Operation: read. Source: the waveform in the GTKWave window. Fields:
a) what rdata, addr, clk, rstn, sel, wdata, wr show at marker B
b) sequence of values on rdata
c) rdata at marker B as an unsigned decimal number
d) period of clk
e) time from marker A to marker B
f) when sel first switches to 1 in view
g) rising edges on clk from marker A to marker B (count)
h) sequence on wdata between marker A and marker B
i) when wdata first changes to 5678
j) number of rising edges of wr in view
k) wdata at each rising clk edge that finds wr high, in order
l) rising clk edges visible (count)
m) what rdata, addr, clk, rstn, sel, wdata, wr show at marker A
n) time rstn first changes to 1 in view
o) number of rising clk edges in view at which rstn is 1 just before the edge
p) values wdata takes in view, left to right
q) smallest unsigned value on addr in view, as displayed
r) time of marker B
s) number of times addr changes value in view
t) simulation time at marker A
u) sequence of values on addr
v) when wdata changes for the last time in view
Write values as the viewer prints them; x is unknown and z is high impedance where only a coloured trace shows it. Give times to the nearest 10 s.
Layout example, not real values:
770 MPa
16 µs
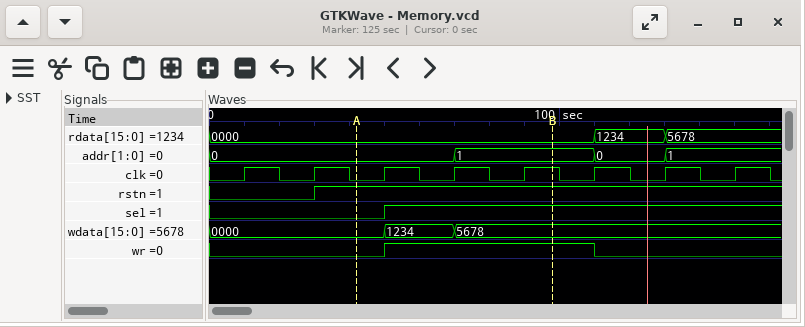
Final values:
rdata=0000, addr=1, clk=1, rstn=1, sel=1, wdata=5678, wr=1
0000, 1234, 5678
0
20 s
60 s
50 s
3
0000, 1234, 5678
70 s
1
1234, 5678, 5678
8
rdata=0000, addr=0, clk=0, rstn=1, sel=0, wdata=0000, wr=0
30 s
6
0000, 1234, 5678
0
100 s
3
40 s
0, 1, 0, 1
70 s
